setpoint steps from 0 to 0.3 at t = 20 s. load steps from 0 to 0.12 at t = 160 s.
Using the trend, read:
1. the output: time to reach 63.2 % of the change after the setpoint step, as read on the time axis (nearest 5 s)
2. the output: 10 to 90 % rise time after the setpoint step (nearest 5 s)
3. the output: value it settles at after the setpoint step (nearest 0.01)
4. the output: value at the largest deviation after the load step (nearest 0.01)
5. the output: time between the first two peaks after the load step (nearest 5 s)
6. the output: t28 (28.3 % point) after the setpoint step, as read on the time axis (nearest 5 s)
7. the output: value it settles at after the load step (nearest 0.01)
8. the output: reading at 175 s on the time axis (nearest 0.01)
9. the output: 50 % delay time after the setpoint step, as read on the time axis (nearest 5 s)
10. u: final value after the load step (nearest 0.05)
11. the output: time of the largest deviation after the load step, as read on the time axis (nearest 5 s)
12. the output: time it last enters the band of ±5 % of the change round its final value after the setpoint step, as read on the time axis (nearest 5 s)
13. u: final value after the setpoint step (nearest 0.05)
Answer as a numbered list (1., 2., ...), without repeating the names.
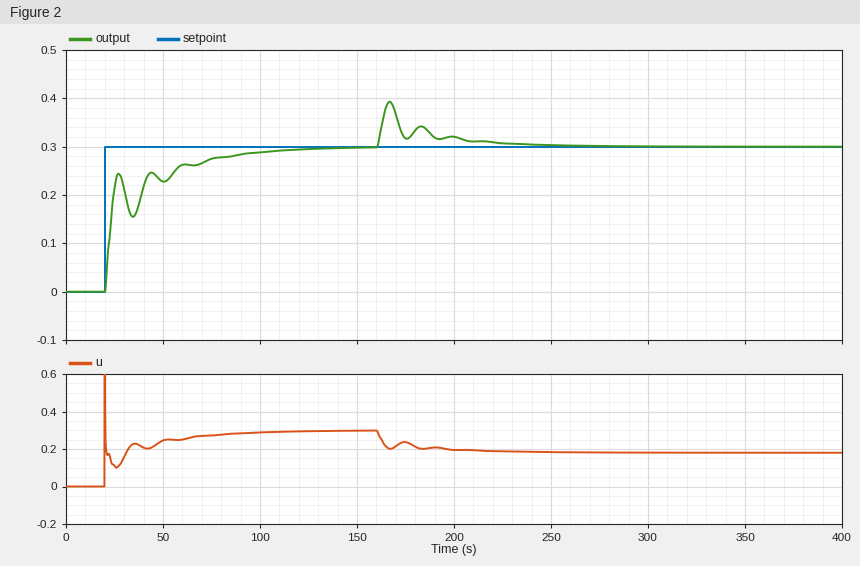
1. 25 s
2. 50 s
3. 0.30
4. 0.39
5. 15 s
6. 20 s
7. 0.30
8. 0.32
9. 25 s
10. 0.20
11. 165 s
12. 90 s
13. 0.30
